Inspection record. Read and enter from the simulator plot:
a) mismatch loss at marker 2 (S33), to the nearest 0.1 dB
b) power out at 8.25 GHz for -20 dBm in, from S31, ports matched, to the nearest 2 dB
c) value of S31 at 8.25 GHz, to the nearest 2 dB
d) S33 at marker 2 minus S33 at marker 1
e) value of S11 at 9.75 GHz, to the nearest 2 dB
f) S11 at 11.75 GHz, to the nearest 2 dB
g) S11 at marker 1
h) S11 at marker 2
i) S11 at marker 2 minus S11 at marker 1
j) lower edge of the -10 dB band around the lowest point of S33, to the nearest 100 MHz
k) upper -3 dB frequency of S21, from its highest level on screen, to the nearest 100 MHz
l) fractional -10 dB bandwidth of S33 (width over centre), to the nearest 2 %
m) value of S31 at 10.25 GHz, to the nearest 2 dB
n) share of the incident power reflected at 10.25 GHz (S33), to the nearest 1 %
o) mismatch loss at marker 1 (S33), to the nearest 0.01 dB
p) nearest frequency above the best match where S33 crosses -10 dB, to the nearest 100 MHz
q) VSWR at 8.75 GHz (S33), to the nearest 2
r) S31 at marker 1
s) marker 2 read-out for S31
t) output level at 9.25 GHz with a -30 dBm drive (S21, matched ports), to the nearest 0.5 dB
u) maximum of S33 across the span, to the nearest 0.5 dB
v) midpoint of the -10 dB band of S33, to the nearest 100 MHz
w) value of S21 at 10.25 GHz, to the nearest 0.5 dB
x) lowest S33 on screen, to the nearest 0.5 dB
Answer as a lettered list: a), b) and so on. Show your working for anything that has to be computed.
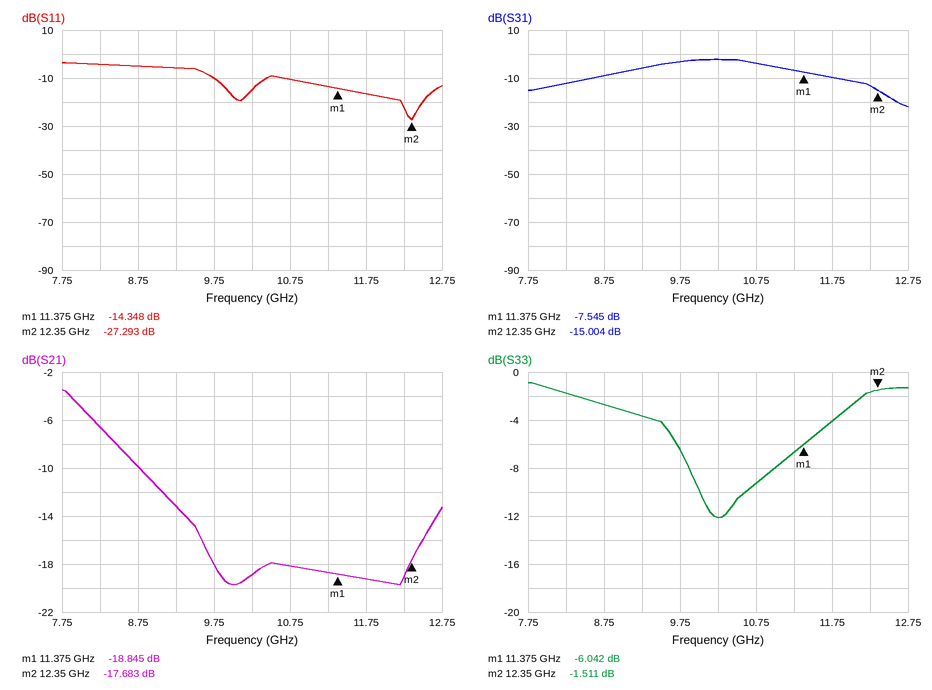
a) −10 log10(1 − 10^(-1.511/10)) ≈ 5.3 dB
b) -20 dBm + (-12 dB) = -32 dBm
c) -12 dB
d) -1.511 − (-6.042) = 4.531 dB
e) -10 dB
f) -16 dB
g) -14.348 dB
h) -27.293 dB
i) -27.293 − (-14.348) = -12.945 dB
j) 10.0 GHz
k) 8.2 GHz
l) 600 MHz / 10.3 GHz ≈ 6 %
m) -2 dB
n) 10^(-12/10) ≈ 6 %
o) −10 log10(1 − 10^(-6.042/10)) ≈ 1.24 dB
p) 10.6 GHz
q) |Γ| = 10^(-2.5/20) = 0.7499; VSWR = (1 + 0.7499)/(1 − 0.7499) ≈ 7.00, so 6 to the nearest 2
r) -7.545 dB
s) -15.004 dB
t) -30 dBm + (-13.0 dB) = -43.0 dBm
u) -1.0 dB
v) 10.3 GHz
w) -19.0 dB
x) -12.0 dB
